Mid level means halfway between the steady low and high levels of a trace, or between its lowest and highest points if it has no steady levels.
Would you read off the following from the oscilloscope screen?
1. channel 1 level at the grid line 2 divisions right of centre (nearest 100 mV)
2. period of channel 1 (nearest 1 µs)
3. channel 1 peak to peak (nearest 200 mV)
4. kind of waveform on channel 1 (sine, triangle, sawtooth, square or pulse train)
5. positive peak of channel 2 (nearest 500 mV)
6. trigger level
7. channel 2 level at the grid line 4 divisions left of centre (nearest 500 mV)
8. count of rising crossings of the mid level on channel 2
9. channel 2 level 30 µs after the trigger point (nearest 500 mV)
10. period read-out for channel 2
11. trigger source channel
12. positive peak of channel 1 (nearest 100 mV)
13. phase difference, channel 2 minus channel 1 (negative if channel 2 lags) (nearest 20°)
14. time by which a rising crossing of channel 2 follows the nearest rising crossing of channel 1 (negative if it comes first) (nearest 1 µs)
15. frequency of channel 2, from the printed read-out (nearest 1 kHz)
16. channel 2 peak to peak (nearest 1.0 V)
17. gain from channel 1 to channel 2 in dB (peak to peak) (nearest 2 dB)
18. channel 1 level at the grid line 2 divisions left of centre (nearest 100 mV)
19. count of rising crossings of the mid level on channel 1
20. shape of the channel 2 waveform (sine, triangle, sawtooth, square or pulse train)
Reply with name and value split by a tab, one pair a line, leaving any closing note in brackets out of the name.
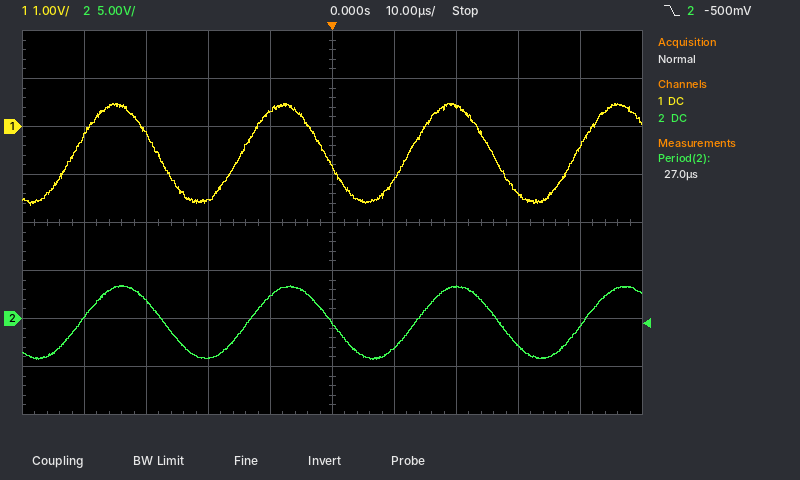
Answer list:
channel 1 level at the grid line 2 divisions right of centre	400 mV
period of channel 1	27 µs
channel 1 peak to peak	2.2 V
kind of waveform on channel 1	sine
positive peak of channel 2	3.5 V
trigger level	-500 mV
channel 2 level at the grid line 4 divisions left of centre	0.0 V
count of rising crossings of the mid level on channel 2	4
channel 2 level 30 µs after the trigger point	-3.0 V
period read-out for channel 2	27.0 µs
trigger source channel	channel 2
positive peak of channel 1	500 mV
phase difference, channel 2 minus channel 1 (negative if channel 2 lags)	-20°
time by which a rising crossing of channel 2 follows the nearest rising crossing of channel 1 (negative if it comes first)	+1 µs
frequency of channel 2, from the printed read-out	37 kHz
channel 2 peak to peak	8.0 V
gain from channel 1 to channel 2 in dB (peak to peak)	12 dB
channel 1 level at the grid line 2 divisions left of centre	-1.5 V
count of rising crossings of the mid level on channel 1	4
shape of the channel 2 waveform	sine
